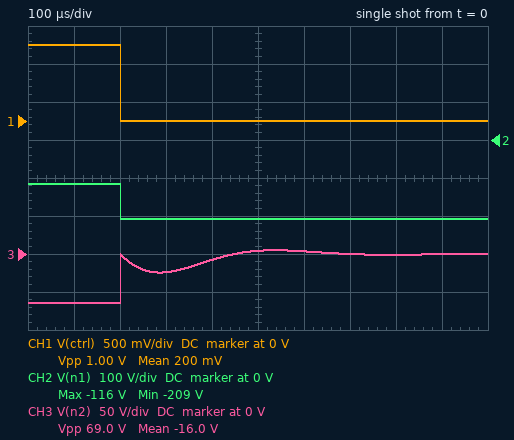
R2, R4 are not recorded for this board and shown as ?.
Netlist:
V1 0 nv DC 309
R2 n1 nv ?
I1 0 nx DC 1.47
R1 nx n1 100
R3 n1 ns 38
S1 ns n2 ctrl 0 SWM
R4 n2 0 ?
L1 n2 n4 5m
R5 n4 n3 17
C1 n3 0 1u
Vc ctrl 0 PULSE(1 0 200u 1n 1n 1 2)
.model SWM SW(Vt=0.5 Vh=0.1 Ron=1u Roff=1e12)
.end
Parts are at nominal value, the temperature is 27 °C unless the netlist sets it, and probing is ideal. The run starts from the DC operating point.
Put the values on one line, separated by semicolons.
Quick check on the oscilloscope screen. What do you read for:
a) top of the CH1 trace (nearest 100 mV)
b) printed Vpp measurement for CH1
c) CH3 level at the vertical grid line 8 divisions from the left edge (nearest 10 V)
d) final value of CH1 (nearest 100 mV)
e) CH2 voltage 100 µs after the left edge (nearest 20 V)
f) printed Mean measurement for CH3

1.0 V; 1.00 V; 0 V; 0 V; -120 V; -16.0 V
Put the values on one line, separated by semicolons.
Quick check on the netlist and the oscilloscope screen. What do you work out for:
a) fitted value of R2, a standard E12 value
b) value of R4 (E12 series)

68 Ω; 47 Ω
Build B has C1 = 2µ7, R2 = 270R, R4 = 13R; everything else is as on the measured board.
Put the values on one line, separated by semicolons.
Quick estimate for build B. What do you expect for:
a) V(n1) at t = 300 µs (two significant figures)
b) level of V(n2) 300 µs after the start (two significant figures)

88 V; 610 mV
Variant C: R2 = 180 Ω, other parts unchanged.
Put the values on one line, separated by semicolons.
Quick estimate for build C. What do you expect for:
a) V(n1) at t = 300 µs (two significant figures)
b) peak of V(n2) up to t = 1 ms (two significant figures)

-44 V; 610 mV
